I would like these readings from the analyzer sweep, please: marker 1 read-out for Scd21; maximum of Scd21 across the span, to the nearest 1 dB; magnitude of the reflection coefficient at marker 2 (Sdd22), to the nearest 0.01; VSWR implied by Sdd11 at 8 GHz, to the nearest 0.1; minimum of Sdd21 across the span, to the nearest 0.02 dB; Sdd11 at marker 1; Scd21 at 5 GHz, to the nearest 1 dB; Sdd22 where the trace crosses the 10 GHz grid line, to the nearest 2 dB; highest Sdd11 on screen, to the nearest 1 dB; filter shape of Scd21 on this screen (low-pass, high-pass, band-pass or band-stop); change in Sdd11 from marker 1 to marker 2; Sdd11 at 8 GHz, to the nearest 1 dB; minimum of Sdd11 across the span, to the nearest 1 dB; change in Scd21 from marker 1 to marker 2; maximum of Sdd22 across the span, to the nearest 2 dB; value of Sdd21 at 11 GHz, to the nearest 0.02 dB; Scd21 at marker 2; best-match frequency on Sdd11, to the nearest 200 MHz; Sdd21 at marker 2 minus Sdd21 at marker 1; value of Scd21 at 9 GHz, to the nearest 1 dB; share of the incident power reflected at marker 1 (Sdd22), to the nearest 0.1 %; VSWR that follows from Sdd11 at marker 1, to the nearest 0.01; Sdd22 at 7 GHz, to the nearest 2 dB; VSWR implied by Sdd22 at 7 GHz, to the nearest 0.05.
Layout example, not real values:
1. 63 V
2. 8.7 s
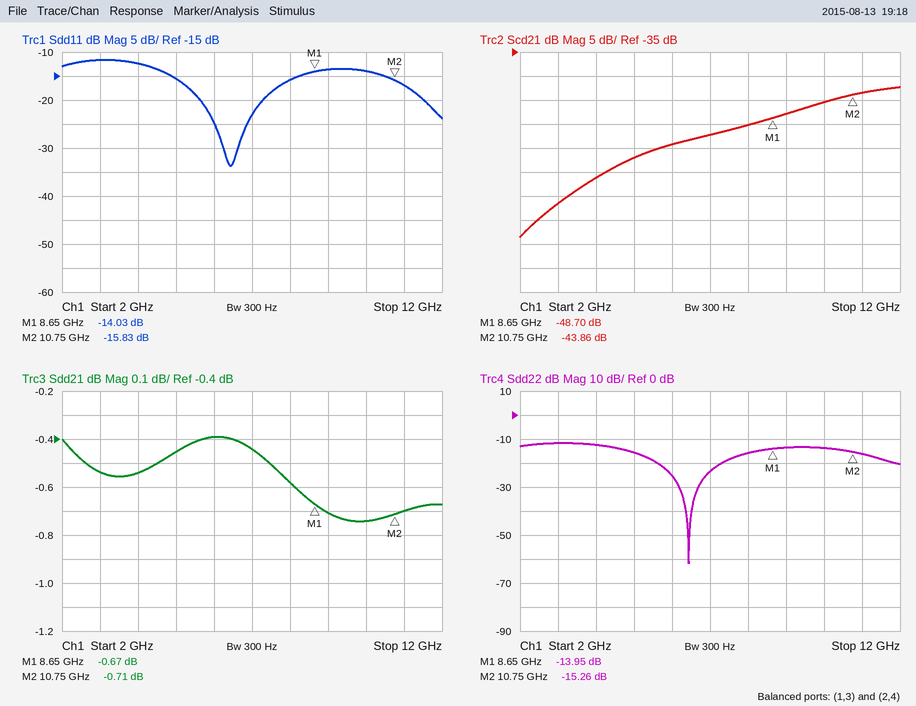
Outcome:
1. -48.70 dB
2. -42 dB
3. 0.17
4. 1.4
5. -0.74 dB
6. -14.03 dB
7. -57 dB
8. -14 dB
9. -12 dB
10. high-pass
11. -1.80 dB
12. -16 dB
13. -34 dB
14. 4.84 dB
15. -12 dB
16. -0.70 dB
17. -43.86 dB
18. 6.4 GHz
19. -0.04 dB
20. -48 dB
21. 4.0 %
22. 1.50
23. -24 dB
24. 1.15
